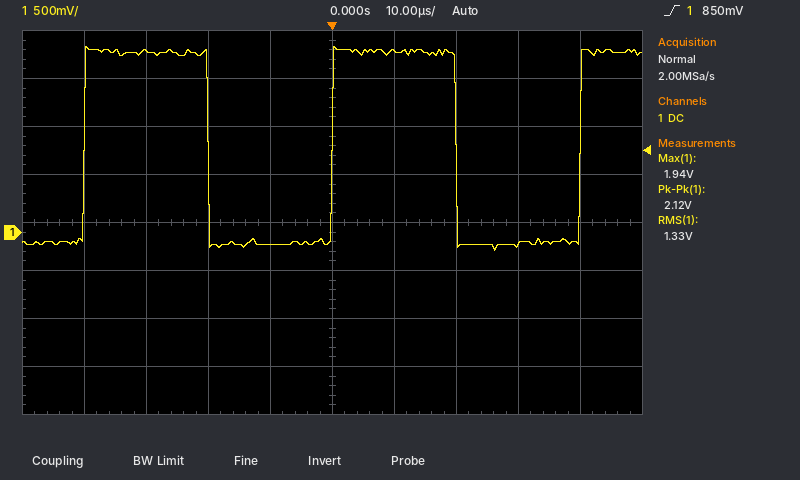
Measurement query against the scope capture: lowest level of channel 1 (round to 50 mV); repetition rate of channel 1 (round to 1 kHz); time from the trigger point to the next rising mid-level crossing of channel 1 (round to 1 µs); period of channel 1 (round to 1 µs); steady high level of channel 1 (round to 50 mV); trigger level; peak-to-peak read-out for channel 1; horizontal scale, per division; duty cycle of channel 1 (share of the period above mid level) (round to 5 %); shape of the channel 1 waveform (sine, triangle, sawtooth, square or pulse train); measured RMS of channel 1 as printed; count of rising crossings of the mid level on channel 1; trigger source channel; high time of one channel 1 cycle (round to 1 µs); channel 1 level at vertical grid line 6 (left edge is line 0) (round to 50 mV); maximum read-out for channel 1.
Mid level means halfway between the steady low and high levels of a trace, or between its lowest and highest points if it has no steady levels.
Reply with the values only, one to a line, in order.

-200 mV
25 kHz
40 µs
40 µs
1.90 V
850 mV
2.12 V
10 µs
50 %
square
1.33 V
3
channel 1
20 µs
1.90 V
1.94 V
